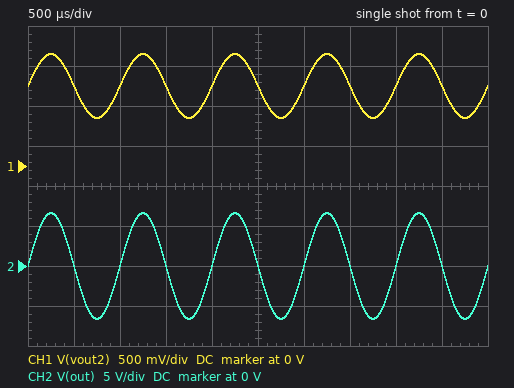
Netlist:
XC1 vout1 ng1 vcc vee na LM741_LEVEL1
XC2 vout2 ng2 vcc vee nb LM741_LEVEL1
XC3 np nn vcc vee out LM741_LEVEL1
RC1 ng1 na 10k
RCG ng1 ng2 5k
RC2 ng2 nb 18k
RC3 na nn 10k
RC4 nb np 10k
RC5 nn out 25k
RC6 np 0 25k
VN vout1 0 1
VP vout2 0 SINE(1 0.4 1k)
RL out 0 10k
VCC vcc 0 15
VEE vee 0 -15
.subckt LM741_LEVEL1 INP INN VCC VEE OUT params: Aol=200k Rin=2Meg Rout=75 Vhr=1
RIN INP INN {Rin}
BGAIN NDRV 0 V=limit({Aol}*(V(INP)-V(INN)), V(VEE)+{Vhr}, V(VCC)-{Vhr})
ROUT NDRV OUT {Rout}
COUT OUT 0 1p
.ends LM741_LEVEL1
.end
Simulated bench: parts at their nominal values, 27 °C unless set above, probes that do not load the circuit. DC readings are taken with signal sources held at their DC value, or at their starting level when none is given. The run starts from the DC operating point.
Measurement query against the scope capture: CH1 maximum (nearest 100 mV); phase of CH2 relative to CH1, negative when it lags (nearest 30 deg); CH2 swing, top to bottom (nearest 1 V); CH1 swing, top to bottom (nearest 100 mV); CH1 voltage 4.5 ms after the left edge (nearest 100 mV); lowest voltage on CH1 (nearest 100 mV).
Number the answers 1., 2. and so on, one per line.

1. 1.4 V
2. 0 deg
3. 13 V
4. 800 mV
5. 1.0 V
6. 600 mV
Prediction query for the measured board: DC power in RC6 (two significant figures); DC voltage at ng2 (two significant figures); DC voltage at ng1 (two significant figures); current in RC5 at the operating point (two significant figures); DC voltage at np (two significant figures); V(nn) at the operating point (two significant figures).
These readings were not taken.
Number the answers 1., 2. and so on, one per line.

1. 20 µW
2. 1.0 V
3. 1.0 V
4. 29 µA
5. 710 mV
6. 710 mV
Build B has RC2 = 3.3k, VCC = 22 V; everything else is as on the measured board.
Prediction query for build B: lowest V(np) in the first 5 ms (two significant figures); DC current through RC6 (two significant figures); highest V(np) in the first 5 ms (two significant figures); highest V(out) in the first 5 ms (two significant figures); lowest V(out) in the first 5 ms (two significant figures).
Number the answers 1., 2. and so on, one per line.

1. 240 mV
2. 29 µA
3. 1.2 V
4. 3.7 V
5. -3.7 V
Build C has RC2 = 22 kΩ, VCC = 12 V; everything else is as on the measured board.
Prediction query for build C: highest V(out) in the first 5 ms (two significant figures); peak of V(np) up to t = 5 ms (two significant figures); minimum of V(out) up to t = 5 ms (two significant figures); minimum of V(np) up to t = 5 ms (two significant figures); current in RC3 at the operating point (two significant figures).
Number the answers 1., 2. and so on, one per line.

1. 7.4 V
2. 2.3 V
3. -7.4 V
4. -830 mV
5. 29 µA
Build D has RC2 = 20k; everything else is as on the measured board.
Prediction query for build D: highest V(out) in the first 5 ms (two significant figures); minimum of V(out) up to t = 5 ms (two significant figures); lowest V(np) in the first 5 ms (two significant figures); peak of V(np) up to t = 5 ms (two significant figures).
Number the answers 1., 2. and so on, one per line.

1. 7.0 V
2. -7.0 V
3. -710 mV
4. 2.1 V
